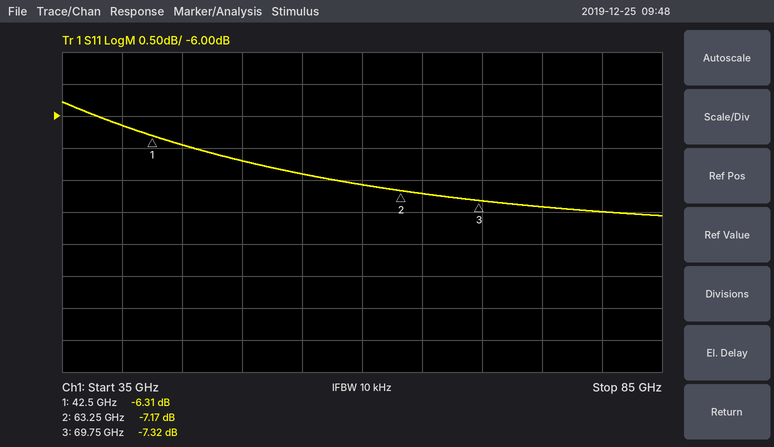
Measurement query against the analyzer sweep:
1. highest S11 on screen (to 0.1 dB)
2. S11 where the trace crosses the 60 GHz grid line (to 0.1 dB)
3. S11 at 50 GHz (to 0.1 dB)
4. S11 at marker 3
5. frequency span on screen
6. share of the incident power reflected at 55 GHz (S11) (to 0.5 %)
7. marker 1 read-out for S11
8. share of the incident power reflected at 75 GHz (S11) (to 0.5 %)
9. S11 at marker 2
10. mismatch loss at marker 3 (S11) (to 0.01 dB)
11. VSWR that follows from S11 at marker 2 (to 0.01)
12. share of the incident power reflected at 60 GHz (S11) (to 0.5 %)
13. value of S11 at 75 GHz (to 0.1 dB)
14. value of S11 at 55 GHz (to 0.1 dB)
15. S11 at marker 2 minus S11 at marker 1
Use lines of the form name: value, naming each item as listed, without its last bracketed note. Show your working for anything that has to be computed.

highest S11 on screen: -5.8 dB
S11 where the trace crosses the 60 GHz grid line: -7.1 dB
S11 at 50 GHz: -6.7 dB
S11 at marker 3: -7.32 dB
frequency span on screen: 50 GHz
share of the incident power reflected at 55 GHz (S11): 10^(-6.9/10) ≈ 20.4 %, so 20.5 % to the nearest 0.5 %
marker 1 read-out for S11: -6.31 dB
share of the incident power reflected at 75 GHz (S11): 10^(-7.4/10) ≈ 18.2 %, so 18.0 % to the nearest 0.5 %
S11 at marker 2: -7.17 dB
mismatch loss at marker 3 (S11): −10 log10(1 − 10^(-7.32/10)) ≈ 0.89 dB
VSWR that follows from S11 at marker 2: (1 + 0.4380)/(1 − 0.4380) ≈ 2.56
share of the incident power reflected at 60 GHz (S11): 10^(-7.1/10) ≈ 19.5 %
value of S11 at 75 GHz: -7.4 dB
value of S11 at 55 GHz: -6.9 dB
S11 at marker 2 minus S11 at marker 1: -7.17 − (-6.31) = -0.86 dB
